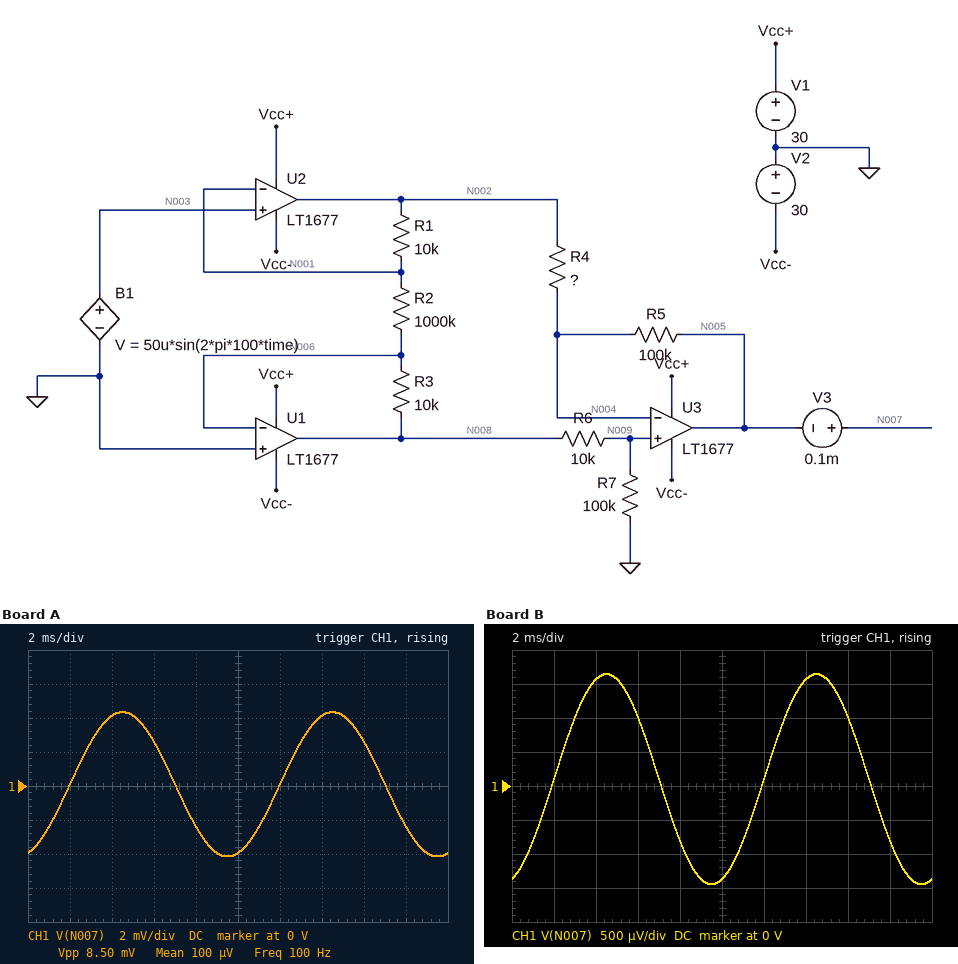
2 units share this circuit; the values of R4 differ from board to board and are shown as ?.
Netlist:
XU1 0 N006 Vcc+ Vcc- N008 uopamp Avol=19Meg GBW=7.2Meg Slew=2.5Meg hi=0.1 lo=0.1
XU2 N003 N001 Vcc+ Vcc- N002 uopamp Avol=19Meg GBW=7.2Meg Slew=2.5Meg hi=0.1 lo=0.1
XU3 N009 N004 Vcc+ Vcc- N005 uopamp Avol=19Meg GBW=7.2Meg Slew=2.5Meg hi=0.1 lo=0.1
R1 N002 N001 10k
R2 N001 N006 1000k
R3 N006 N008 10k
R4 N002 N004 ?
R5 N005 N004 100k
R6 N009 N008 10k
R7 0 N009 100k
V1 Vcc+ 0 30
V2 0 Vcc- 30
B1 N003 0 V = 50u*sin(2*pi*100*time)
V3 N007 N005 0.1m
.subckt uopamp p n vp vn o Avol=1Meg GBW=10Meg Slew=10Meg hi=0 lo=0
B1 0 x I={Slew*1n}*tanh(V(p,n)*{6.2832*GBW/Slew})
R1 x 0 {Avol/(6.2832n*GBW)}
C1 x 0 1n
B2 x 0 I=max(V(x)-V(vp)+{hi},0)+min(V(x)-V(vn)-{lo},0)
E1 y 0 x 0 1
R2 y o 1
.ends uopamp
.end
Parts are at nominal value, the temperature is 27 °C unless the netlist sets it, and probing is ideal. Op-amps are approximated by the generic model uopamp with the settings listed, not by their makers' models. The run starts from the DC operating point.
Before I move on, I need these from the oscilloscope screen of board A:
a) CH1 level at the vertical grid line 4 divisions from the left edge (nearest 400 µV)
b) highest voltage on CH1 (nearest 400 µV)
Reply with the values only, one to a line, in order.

-2.4 mV
4.4 mV
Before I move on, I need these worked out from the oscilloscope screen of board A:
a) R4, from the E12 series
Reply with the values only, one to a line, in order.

1.2 kΩ
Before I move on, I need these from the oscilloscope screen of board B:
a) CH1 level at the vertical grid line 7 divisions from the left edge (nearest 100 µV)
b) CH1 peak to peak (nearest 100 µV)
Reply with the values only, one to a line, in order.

1.6 mV
3.1 mV
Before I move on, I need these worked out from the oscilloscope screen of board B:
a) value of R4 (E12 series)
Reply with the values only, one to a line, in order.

3.3 kΩ
